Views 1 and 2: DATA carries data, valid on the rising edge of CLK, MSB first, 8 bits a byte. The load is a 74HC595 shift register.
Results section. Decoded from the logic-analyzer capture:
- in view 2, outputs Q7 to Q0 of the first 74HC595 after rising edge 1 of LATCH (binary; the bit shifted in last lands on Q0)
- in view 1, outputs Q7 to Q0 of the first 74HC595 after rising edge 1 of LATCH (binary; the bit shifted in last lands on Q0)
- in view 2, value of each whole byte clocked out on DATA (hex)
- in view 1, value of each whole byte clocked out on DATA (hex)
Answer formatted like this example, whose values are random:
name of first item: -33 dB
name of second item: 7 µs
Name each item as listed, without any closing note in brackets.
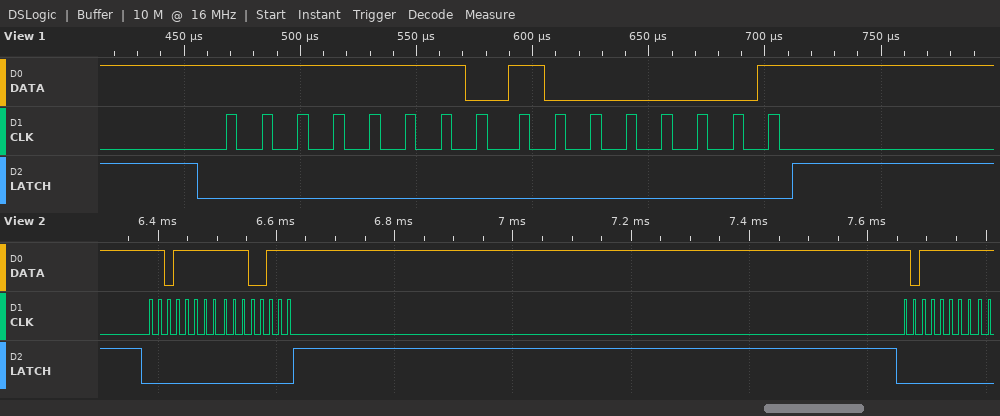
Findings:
in view 2, outputs Q7 to Q0 of the first 74HC595 after rising edge 1 of LATCH: 11100111
in view 1, outputs Q7 to Q0 of the first 74HC595 after rising edge 1 of LATCH: 10000001
in view 2, value of each whole byte clocked out on DATA: DF E7 BF
in view 1, value of each whole byte clocked out on DATA: FE 81
